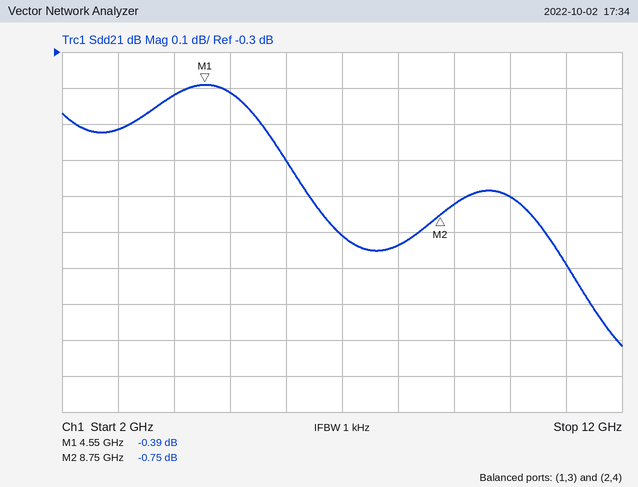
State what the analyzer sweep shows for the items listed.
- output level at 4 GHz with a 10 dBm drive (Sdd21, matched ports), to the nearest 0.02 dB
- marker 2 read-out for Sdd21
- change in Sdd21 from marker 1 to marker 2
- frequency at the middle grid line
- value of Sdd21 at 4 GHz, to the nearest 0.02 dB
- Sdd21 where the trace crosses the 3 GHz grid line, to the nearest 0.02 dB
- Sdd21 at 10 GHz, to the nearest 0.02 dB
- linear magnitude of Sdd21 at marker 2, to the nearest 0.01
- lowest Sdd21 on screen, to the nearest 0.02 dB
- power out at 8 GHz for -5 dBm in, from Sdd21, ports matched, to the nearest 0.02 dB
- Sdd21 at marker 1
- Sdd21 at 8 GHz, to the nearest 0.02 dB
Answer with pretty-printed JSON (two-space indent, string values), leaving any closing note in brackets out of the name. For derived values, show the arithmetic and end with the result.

{
  "output level at 4 GHz with a 10 dBm drive (Sdd21, matched ports), to the nearest 0.02 dB": "10 dBm + (-0.42 dB) = 9.58 dBm",
  "marker 2 read-out for Sdd21": "-0.75 dB",
  "change in Sdd21 from marker 1 to marker 2": "-0.75 − (-0.39) = -0.36 dB",
  "frequency at the middle grid line": "7 GHz",
  "value of Sdd21 at 4 GHz, to the nearest 0.02 dB": "-0.42 dB",
  "Sdd21 where the trace crosses the 3 GHz grid line, to the nearest 0.02 dB": "-0.52 dB",
  "Sdd21 at 10 GHz, to the nearest 0.02 dB": "-0.70 dB",
  "linear magnitude of Sdd21 at marker 2, to the nearest 0.01": "10^(-0.75/20) ≈ 0.92",
  "lowest Sdd21 on screen, to the nearest 0.02 dB": "-1.12 dB",
  "power out at 8 GHz for -5 dBm in, from Sdd21, ports matched, to the nearest 0.02 dB": "-5 dBm + (-0.84 dB) = -5.84 dBm",
  "Sdd21 at marker 1": "-0.39 dB",
  "Sdd21 at 8 GHz, to the nearest 0.02 dB": "-0.84 dB"
}
